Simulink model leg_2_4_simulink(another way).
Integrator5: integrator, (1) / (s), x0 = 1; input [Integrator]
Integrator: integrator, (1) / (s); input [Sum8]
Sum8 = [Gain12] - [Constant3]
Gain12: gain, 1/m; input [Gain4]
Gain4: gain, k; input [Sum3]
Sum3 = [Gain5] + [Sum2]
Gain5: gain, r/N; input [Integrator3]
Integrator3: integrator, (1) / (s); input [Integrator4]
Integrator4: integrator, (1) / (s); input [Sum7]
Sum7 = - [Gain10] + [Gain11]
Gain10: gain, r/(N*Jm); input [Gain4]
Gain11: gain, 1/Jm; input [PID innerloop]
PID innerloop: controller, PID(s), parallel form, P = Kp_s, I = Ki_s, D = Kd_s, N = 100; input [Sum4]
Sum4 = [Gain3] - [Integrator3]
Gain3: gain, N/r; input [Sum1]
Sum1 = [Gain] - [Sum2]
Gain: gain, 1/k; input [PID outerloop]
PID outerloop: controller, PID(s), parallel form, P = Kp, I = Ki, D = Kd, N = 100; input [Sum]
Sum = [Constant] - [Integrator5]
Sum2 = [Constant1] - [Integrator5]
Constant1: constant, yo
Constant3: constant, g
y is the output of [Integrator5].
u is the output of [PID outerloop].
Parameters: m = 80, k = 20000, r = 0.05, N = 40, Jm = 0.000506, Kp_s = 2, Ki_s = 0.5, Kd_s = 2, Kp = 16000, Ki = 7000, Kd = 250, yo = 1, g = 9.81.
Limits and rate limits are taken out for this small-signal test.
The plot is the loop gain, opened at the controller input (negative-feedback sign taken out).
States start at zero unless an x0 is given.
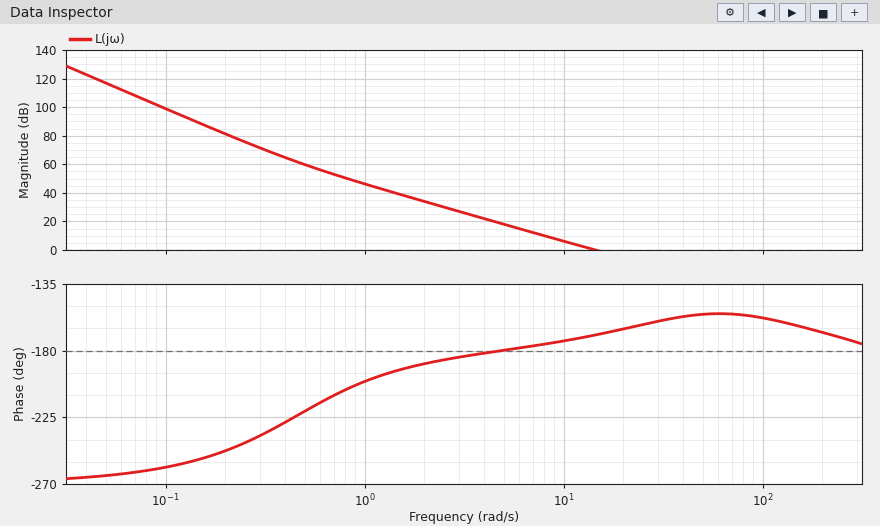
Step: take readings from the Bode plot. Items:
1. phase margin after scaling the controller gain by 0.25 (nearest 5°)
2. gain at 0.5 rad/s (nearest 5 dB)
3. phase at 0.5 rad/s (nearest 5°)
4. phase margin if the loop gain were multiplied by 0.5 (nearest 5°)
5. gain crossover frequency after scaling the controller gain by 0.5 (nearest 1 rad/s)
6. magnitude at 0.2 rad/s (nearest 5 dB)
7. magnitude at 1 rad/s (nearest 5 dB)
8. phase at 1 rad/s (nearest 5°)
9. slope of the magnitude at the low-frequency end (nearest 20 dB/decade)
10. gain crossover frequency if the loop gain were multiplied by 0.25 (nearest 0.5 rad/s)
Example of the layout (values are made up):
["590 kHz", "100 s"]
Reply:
["5°", "60 dB", "-220°", "5°", "10 rad/s", "80 dB", "45 dB", "-200°", "-60 dB/decade", "7.0 rad/s"]
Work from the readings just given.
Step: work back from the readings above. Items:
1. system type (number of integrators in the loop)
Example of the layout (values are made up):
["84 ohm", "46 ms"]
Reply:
["3"]
